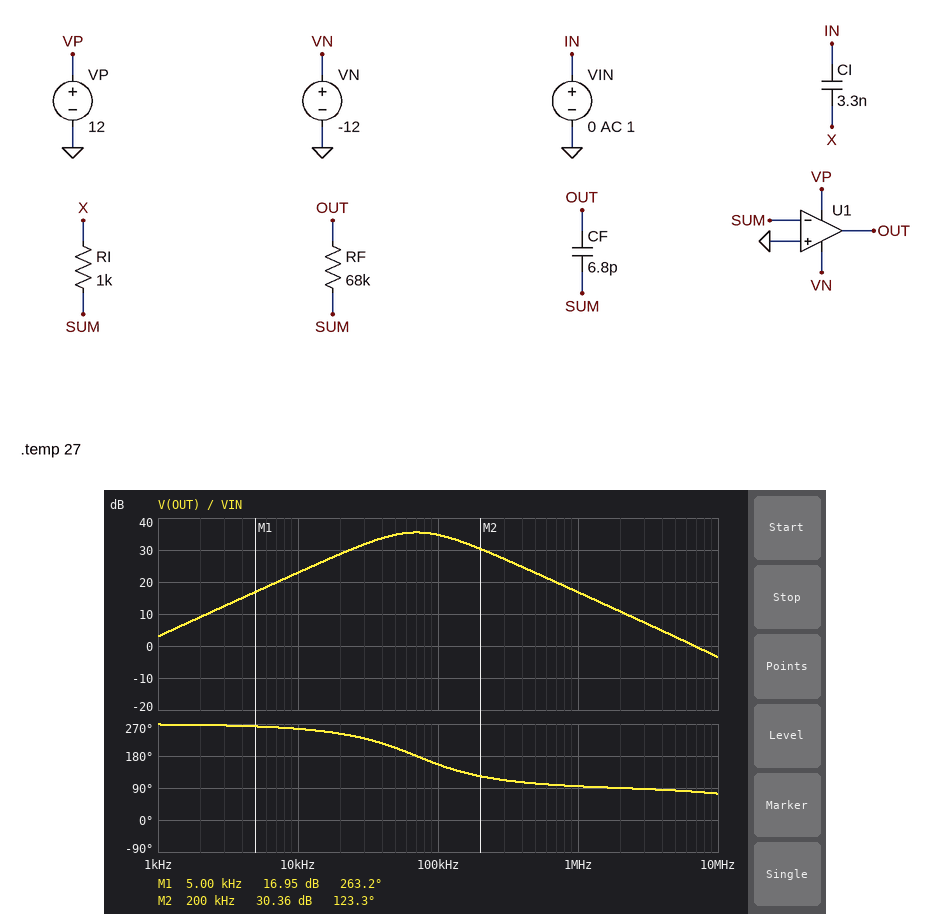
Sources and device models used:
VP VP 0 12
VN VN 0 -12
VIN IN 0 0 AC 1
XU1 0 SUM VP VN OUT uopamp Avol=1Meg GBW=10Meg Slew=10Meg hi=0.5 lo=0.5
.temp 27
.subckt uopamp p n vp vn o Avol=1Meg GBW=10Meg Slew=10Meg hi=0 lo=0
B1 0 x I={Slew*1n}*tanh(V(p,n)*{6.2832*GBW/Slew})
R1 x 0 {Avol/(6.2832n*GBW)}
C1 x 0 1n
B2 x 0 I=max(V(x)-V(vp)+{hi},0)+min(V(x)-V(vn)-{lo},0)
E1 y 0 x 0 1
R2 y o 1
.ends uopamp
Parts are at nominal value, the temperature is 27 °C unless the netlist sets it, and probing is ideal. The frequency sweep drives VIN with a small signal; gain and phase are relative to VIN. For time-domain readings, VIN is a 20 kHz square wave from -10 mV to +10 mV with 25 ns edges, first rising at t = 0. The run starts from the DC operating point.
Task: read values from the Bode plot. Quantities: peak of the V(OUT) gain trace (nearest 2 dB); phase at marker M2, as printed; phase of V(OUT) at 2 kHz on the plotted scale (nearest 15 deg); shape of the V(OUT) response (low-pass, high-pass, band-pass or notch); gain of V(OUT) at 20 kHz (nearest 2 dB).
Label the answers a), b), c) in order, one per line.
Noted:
a) 36 dB
b) 123.3 deg
c) 270 deg
d) band-pass
e) 28 dB
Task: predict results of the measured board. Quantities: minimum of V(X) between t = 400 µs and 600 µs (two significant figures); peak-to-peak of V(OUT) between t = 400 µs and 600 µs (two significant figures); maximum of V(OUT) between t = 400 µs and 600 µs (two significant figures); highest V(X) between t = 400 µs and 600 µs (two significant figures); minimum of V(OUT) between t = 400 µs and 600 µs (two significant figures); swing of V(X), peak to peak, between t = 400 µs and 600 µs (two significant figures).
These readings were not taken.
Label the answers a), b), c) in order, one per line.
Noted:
a) -20 mV
b) 1.6 V
c) 820 mV
d) 20 mV
e) -820 mV
f) 40 mV
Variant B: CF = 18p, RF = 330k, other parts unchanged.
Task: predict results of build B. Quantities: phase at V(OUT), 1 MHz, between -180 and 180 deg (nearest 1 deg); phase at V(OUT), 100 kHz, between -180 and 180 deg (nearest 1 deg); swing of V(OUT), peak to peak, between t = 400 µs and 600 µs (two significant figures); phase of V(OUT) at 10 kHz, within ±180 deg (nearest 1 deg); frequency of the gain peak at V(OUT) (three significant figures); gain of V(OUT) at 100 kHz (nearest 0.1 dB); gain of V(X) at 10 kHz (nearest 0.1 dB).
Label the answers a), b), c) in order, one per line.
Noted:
a) 89 deg
b) 113 deg
c) 3.2 V
d) -124 deg
e) 26.2 kHz
f) 33.3 dB
g) -12.2 dB
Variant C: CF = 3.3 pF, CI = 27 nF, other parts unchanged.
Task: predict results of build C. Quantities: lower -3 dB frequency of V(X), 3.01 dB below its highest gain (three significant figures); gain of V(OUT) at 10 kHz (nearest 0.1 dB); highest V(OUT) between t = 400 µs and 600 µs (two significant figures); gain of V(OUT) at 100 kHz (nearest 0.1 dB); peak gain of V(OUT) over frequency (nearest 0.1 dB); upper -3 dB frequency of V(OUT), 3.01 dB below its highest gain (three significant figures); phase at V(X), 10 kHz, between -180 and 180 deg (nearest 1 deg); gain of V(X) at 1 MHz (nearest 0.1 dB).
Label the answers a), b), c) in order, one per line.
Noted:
a) 5.99 kHz
b) 35.6 dB
c) 860 mV
d) 34.6 dB
e) 36.6 dB
f) 127 kHz
g) 31 deg
h) 0 dB
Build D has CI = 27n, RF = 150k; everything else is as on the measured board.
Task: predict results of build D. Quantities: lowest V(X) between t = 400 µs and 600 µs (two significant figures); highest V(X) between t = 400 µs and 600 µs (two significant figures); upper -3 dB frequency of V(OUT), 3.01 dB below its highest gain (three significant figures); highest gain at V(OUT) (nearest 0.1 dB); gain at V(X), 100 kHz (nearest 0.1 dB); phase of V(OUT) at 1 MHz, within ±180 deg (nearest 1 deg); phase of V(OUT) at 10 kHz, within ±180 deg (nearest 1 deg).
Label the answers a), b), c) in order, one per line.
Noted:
a) -14 mV
b) 14 mV
c) 53.5 kHz
d) 43.2 dB
e) 0.1 dB
f) 91 deg
g) -160 deg
